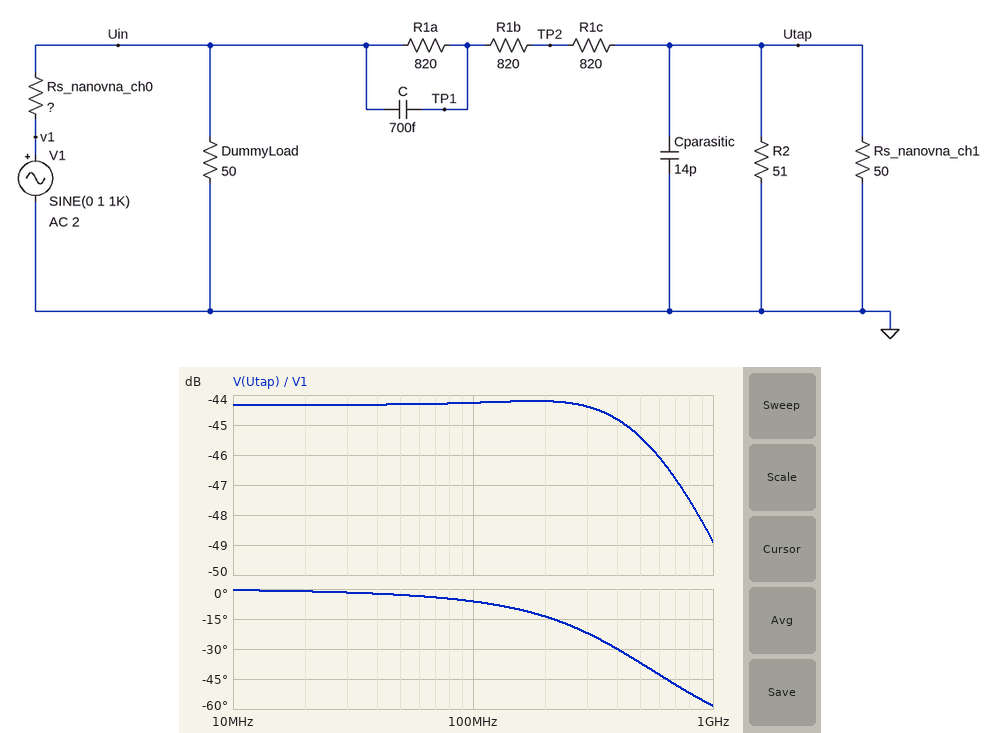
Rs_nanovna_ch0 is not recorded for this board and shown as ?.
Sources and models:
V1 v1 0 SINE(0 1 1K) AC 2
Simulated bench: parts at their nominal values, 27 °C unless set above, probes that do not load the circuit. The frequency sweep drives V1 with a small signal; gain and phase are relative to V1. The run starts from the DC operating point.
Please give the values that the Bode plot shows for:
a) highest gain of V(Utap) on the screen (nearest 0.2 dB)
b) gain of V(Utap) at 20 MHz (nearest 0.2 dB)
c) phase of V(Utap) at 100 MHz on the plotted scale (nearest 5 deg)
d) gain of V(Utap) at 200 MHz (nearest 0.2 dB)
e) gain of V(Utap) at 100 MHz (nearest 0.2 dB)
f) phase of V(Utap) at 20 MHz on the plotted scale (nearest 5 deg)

-44.2 dB
-44.4 dB
-5 deg
-44.2 dB
-44.2 dB
0 deg
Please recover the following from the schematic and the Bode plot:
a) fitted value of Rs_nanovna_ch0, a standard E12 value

33 Ω
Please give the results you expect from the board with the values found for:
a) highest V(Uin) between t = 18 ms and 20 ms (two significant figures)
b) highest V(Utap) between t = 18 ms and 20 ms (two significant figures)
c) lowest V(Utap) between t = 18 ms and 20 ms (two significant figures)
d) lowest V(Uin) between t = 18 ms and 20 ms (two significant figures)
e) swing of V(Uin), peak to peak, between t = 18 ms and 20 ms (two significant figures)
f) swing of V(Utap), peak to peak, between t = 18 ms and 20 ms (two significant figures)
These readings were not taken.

600 mV
6.1 mV
-6.1 mV
-600 mV
1.2 V
12 mV
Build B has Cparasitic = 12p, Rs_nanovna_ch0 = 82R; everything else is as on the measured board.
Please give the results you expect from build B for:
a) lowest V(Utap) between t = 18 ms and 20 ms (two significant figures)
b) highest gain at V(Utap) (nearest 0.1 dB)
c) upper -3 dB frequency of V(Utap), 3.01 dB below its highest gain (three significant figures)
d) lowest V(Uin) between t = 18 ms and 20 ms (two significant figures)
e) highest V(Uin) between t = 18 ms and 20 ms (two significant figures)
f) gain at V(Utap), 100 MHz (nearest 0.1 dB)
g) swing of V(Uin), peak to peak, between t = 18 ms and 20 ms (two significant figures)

-3.8 mV
-48.1 dB
868 MHz
-370 mV
370 mV
-48.3 dB
750 mV
